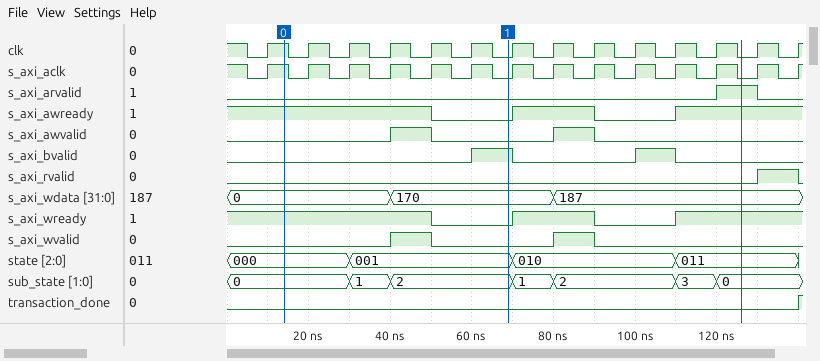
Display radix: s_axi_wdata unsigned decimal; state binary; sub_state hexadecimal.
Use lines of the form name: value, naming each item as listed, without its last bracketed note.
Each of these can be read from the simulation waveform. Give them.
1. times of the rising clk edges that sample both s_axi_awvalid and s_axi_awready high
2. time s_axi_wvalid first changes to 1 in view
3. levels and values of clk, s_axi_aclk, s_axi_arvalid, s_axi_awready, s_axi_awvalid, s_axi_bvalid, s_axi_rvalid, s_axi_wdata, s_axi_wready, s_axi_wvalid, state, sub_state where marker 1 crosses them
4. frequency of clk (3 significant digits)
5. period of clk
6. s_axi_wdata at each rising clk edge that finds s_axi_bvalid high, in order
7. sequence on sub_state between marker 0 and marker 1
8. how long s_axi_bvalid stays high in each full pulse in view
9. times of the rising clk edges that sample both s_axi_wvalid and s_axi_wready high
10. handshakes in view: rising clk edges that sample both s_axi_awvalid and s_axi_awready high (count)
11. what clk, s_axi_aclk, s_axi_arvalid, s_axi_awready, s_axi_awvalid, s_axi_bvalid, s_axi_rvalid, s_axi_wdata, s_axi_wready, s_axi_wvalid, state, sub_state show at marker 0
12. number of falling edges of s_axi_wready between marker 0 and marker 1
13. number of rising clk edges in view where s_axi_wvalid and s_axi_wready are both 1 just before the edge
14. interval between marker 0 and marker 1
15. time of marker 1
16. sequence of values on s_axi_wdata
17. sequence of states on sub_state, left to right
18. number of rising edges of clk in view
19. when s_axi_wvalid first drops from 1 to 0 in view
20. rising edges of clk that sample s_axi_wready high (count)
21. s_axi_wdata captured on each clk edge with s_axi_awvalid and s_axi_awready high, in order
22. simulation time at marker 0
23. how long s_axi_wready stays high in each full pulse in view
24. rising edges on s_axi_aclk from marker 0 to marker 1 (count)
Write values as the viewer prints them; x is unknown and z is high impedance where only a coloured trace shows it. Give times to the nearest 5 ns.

times of the rising clk edges that sample both s_axi_awvalid and s_axi_awready high: 50 ns, 90 ns
time s_axi_wvalid first changes to 1 in view: 40 ns
levels and values of clk, s_axi_aclk, s_axi_arvalid, s_axi_awready, s_axi_awvalid, s_axi_bvalid, s_axi_rvalid, s_axi_wdata, s_axi_wready, s_axi_wvalid, state, sub_state where marker 1 crosses them: clk=0, s_axi_aclk=0, s_axi_arvalid=0, s_axi_awready=0, s_axi_awvalid=0, s_axi_bvalid=1, s_axi_rvalid=0, s_axi_wdata=170, s_axi_wready=0, s_axi_wvalid=0, state=001, sub_state=2
frequency of clk: 100 MHz
period of clk: 10 ns
s_axi_wdata at each rising clk edge that finds s_axi_bvalid high, in order: 170, 187
sequence on sub_state between marker 0 and marker 1: 0, 1, 2
how long s_axi_bvalid stays high in each full pulse in view: 10 ns, 10 ns
times of the rising clk edges that sample both s_axi_wvalid and s_axi_wready high: 50 ns, 90 ns
handshakes in view: rising clk edges that sample both s_axi_awvalid and s_axi_awready high: 2
what clk, s_axi_aclk, s_axi_arvalid, s_axi_awready, s_axi_awvalid, s_axi_bvalid, s_axi_rvalid, s_axi_wdata, s_axi_wready, s_axi_wvalid, state, sub_state show at marker 0: clk=1, s_axi_aclk=1, s_axi_arvalid=0, s_axi_awready=1, s_axi_awvalid=0, s_axi_bvalid=0, s_axi_rvalid=0, s_axi_wdata=0, s_axi_wready=1, s_axi_wvalid=0, state=000, sub_state=0
number of falling edges of s_axi_wready between marker 0 and marker 1: 1
number of rising clk edges in view where s_axi_wvalid and s_axi_wready are both 1 just before the edge: 2
interval between marker 0 and marker 1: 55 ns
time of marker 1: 70 ns
sequence of values on s_axi_wdata: 0, 170, 187
sequence of states on sub_state, left to right: 0, 1, 2, 1, 2, 3, 0
number of rising edges of clk in view: 14
when s_axi_wvalid first drops from 1 to 0 in view: 50 ns
rising edges of clk that sample s_axi_wready high: 10
s_axi_wdata captured on each clk edge with s_axi_awvalid and s_axi_awready high, in order: 170, 187
simulation time at marker 0: 15 ns
how long s_axi_wready stays high in each full pulse in view: 20 ns
rising edges on s_axi_aclk from marker 0 to marker 1: 5
